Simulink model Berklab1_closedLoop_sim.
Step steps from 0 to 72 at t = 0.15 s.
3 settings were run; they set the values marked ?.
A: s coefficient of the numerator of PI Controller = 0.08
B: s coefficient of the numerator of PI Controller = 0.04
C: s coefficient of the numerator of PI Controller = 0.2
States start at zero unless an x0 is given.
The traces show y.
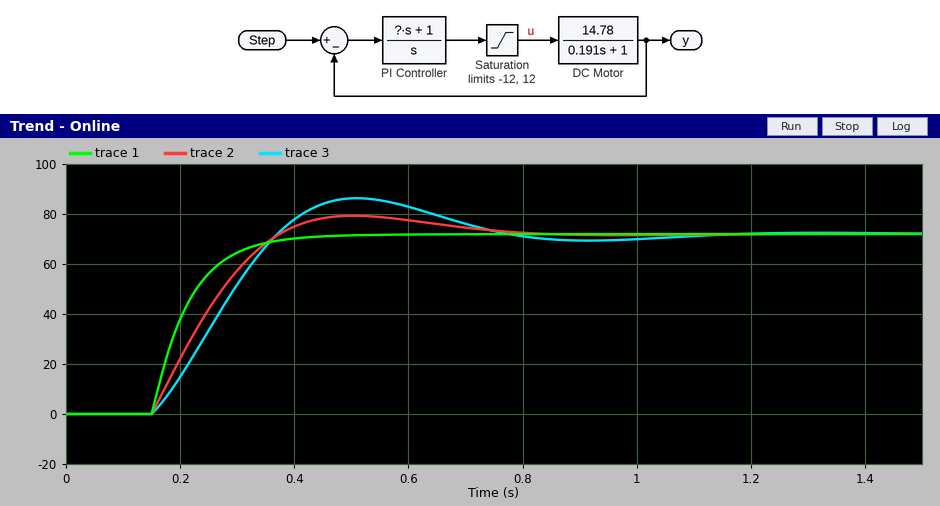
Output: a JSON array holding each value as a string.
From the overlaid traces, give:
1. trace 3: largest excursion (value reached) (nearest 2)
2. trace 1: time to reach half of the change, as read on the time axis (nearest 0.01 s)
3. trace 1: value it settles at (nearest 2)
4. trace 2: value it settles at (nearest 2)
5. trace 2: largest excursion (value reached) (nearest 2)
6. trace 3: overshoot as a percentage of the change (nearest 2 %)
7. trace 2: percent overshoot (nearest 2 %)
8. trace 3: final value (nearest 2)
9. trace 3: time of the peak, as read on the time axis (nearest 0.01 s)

["86", "0.20 s", "72", "72", "80", "20 %", "10 %", "72", "0.51 s"]
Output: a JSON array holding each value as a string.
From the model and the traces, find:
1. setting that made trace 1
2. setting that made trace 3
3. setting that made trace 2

["C", "B", "A"]
